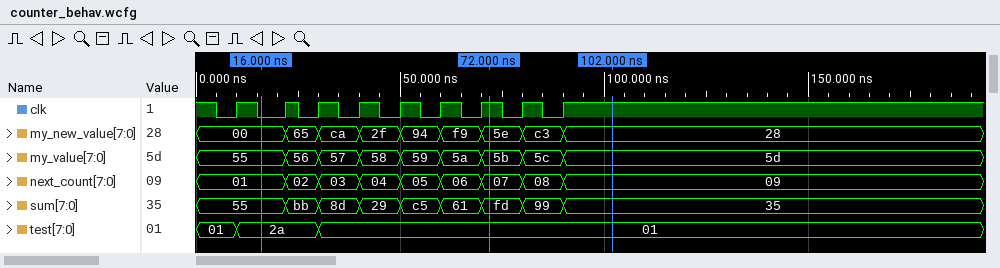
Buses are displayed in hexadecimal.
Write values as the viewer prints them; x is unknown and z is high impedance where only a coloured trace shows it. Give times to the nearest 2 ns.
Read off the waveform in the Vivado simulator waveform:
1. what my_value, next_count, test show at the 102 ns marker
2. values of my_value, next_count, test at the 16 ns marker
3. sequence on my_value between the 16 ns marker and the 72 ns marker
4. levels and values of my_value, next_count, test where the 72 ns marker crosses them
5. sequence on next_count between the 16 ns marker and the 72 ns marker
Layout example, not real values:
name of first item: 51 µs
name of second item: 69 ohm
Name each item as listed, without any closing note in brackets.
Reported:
what my_value, next_count, test show at the 102 ns marker: my_value=5d, next_count=09, test=01
values of my_value, next_count, test at the 16 ns marker: my_value=55, next_count=01, test=2a
sequence on my_value between the 16 ns marker and the 72 ns marker: 55, 56, 57, 58, 59, 5a, 5b
levels and values of my_value, next_count, test where the 72 ns marker crosses them: my_value=5b, next_count=07, test=01
sequence on next_count between the 16 ns marker and the 72 ns marker: 01, 02, 03, 04, 05, 06, 07
